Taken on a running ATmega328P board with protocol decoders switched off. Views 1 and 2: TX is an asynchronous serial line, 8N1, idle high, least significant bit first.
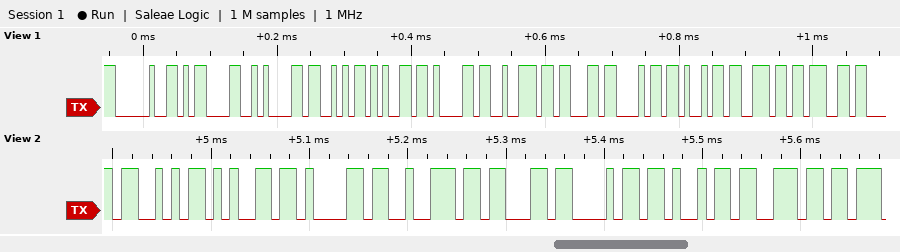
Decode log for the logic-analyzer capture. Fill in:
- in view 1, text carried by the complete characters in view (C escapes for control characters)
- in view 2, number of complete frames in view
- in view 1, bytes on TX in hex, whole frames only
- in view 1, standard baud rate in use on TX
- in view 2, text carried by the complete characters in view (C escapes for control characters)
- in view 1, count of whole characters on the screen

" \r\nSearching"
8
20 0D 0A 53 65 61 72 63 68 69 6E 67
115200 baud
"Searchin"
12
